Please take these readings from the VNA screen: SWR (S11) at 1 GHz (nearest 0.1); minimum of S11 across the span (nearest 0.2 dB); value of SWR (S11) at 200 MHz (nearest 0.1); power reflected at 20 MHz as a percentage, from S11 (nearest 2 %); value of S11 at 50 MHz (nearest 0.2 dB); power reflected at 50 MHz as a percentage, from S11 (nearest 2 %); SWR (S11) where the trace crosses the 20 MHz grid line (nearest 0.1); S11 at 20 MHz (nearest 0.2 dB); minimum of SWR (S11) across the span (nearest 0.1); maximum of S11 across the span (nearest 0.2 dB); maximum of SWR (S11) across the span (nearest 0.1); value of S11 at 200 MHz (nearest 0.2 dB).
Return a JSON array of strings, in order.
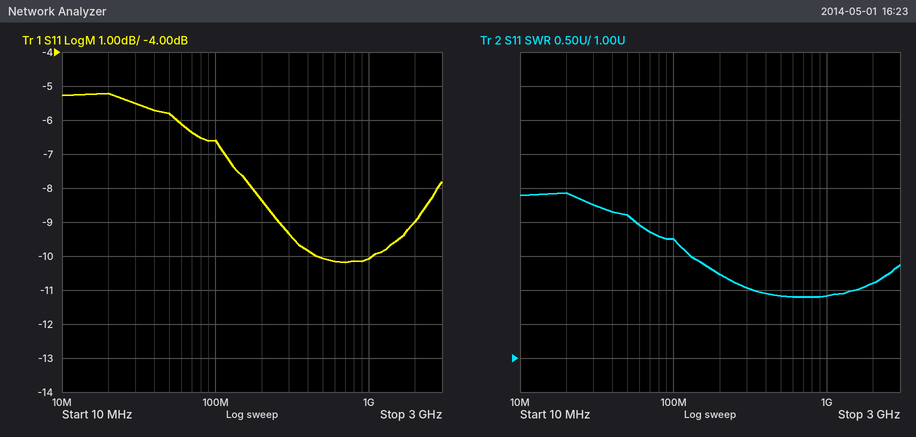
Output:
["1.9", "-10.2 dB", "2.2", "30 %", "-5.8 dB", "26 %", "3.4", "-5.2 dB", "1.9", "-5.2 dB", "3.4", "-8.4 dB"]
